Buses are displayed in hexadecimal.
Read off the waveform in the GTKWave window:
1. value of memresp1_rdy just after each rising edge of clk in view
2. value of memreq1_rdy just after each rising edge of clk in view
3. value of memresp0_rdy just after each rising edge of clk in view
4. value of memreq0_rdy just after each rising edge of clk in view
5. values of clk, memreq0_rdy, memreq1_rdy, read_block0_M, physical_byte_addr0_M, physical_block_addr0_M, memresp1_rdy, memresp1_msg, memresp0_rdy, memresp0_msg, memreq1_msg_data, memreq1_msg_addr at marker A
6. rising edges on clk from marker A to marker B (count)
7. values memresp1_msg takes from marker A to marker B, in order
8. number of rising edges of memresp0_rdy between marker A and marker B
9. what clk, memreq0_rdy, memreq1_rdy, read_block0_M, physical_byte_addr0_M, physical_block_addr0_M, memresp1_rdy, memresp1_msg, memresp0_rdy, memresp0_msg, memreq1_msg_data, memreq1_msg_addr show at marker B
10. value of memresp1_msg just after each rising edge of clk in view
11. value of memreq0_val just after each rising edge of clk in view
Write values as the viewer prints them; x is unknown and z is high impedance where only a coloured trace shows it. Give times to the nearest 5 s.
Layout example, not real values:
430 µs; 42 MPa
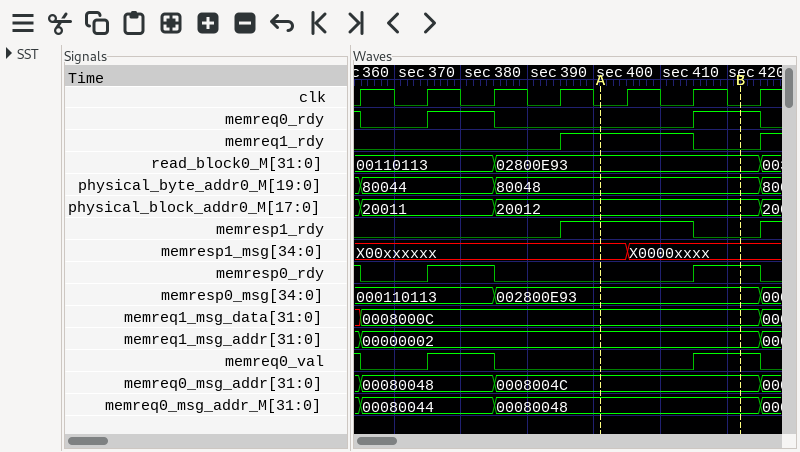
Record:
0 0 0 1 1 0 1; 0 0 0 1 1 0 1; 0 1 0 0 0 1 0; 0 1 0 0 0 1 0; clk=0, memreq0_rdy=0, memreq1_rdy=1, read_block0_M=02800E93, physical_byte_addr0_M=80048, physical_block_addr0_M=20012, memresp1_rdy=1, memresp1_msg=X00xxxxxx, memresp0_rdy=0, memresp0_msg=002800E93, memreq1_msg_data=0008000C, memreq1_msg_addr=00000002; 2; X00xxxxxx, X0000xxxx; 1; clk=0, memreq0_rdy=1, memreq1_rdy=0, read_block0_M=02800E93, physical_byte_addr0_M=80048, physical_block_addr0_M=20012, memresp1_rdy=0, memresp1_msg=X0000xxxx, memresp0_rdy=1, memresp0_msg=002800E93, memreq1_msg_data=0008000C, memreq1_msg_addr=00000002; X00xxxxxx, X00xxxxxx, X00xxxxxx, X00xxxxxx, X0000xxxx, X0000xxxx, X0000xxxx; 0 1 0 0 0 1 0
